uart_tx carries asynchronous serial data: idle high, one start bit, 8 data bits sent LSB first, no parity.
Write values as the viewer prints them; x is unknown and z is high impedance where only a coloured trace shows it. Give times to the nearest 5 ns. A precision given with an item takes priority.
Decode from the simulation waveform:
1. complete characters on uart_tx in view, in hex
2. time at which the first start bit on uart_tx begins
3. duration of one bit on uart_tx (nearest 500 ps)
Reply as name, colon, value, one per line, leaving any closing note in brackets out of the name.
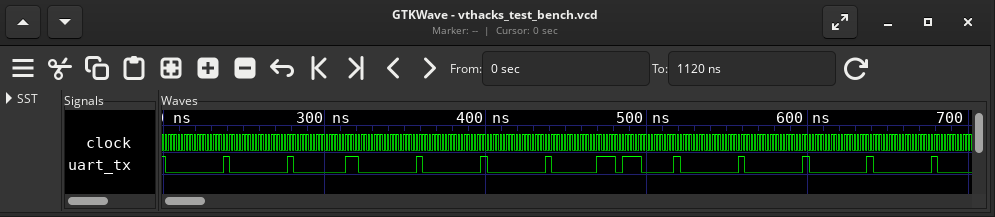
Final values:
complete characters on uart_tx in view, in hex: 00, 00, 80, 00, 00, 00, C0, 07, 00, 00, 00, 00
time at which the first start bit on uart_tx begins: 200 ns
duration of one bit on uart_tx: 4000 ps
